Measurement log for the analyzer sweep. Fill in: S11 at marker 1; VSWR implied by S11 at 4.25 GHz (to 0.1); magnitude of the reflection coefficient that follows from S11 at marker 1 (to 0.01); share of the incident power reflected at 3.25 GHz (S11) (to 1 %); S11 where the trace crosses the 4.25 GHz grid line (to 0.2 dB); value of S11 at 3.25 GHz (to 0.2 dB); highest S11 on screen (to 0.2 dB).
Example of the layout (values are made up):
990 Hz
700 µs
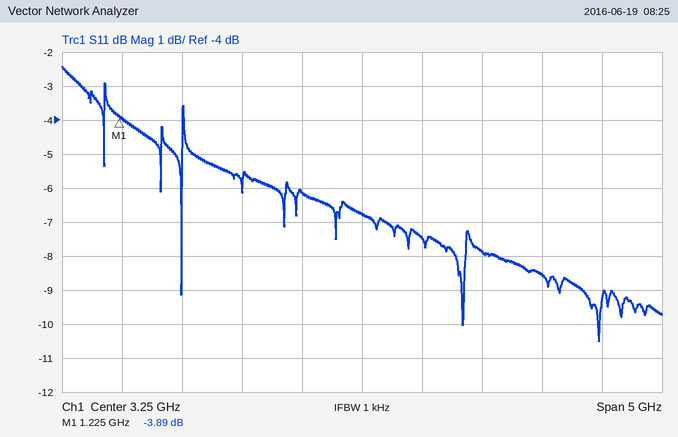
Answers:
-3.89 dB
2.4
0.64
21 %
-7.8 dB
-6.8 dB
-2.4 dB
